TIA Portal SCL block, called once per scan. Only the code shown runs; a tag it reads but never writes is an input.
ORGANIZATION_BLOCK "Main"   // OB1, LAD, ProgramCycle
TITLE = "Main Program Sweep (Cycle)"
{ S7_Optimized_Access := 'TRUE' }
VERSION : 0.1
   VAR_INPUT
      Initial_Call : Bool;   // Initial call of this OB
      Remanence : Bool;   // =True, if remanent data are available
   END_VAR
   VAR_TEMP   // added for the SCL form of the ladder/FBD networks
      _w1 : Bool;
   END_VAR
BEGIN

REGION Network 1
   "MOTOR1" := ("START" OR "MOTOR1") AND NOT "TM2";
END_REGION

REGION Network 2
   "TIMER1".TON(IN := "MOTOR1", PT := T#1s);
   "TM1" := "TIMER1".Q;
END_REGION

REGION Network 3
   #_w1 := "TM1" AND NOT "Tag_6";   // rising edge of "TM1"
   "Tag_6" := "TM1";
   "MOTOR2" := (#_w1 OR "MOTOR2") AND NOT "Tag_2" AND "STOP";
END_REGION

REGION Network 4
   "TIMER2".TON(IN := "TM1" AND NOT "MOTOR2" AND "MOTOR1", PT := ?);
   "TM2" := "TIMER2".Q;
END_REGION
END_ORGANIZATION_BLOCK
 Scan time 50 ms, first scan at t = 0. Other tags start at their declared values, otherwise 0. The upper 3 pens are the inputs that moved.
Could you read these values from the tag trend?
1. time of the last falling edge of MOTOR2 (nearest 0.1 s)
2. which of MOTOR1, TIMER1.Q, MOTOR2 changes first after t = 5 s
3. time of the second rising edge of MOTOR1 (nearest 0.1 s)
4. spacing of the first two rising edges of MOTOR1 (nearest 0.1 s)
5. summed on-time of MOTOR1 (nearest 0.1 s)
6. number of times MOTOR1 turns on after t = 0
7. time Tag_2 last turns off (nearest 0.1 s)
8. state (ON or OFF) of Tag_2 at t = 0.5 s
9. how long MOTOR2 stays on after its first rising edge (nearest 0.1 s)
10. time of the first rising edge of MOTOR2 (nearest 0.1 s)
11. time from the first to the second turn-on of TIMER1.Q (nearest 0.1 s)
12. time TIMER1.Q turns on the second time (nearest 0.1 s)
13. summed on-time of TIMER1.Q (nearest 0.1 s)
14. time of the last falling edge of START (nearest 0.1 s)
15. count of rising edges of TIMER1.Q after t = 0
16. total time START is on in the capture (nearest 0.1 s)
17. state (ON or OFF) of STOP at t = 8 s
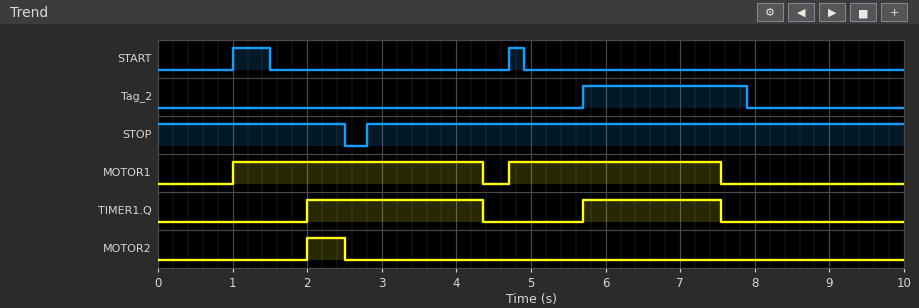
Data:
2.5 s
TIMER1.Q
4.7 s
3.7 s
6.2 s
2
7.9 s
OFF
0.5 s
2.0 s
3.7 s
5.7 s
4.2 s
4.9 s
2
0.7 s
ON
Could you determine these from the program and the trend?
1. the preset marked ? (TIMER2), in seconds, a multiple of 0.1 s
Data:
1.8 s
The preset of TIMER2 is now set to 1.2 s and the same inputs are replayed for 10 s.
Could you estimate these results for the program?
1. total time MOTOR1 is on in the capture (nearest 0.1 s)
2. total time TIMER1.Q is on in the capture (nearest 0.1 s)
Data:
5.0 s
3.0 s
